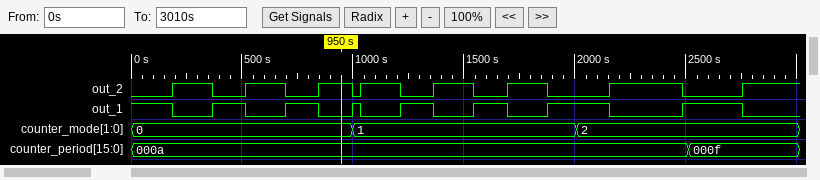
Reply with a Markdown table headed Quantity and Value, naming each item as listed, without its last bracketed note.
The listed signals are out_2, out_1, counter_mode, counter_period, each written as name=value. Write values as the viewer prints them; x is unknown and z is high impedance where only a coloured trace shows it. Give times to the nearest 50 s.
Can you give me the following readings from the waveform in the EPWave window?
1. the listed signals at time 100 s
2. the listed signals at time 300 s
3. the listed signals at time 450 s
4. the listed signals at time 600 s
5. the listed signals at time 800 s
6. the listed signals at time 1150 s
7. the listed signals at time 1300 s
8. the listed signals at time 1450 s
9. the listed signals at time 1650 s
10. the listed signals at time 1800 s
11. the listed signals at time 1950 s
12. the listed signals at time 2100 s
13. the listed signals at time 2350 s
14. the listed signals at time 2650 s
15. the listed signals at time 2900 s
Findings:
| Quantity | Value |
|---|---|
| the listed signals at time 100 s | out_2=0, out_1=1, counter_mode=0, counter_period=000a |
| the listed signals at time 300 s | out_2=1, out_1=0, counter_mode=0, counter_period=000a |
| the listed signals at time 450 s | out_2=0, out_1=1, counter_mode=0, counter_period=000a |
| the listed signals at time 600 s | out_2=1, out_1=0, counter_mode=0, counter_period=000a |
| the listed signals at time 800 s | out_2=0, out_1=1, counter_mode=0, counter_period=000a |
| the listed signals at time 1150 s | out_2=1, out_1=0, counter_mode=1, counter_period=000a |
| the listed signals at time 1300 s | out_2=0, out_1=1, counter_mode=1, counter_period=000a |
| the listed signals at time 1450 s | out_2=1, out_1=0, counter_mode=1, counter_period=000a |
| the listed signals at time 1650 s | out_2=0, out_1=1, counter_mode=1, counter_period=000a |
| the listed signals at time 1800 s | out_2=1, out_1=0, counter_mode=1, counter_period=000a |
| the listed signals at time 1950 s | out_2=0, out_1=1, counter_mode=1, counter_period=000a |
| the listed signals at time 2100 s | out_2=0, out_1=1, counter_mode=2, counter_period=000a |
| the listed signals at time 2350 s | out_2=1, out_1=0, counter_mode=2, counter_period=000a |
| the listed signals at time 2650 s | out_2=0, out_1=1, counter_mode=2, counter_period=000f |
| the listed signals at time 2900 s | out_2=1, out_1=0, counter_mode=2, counter_period=000f |
